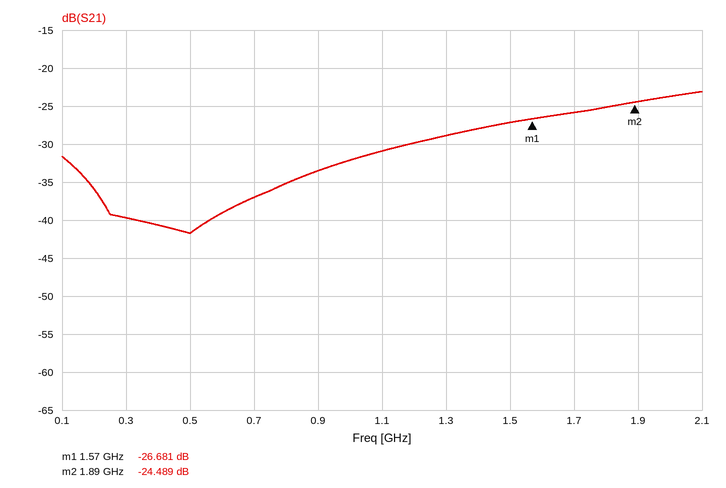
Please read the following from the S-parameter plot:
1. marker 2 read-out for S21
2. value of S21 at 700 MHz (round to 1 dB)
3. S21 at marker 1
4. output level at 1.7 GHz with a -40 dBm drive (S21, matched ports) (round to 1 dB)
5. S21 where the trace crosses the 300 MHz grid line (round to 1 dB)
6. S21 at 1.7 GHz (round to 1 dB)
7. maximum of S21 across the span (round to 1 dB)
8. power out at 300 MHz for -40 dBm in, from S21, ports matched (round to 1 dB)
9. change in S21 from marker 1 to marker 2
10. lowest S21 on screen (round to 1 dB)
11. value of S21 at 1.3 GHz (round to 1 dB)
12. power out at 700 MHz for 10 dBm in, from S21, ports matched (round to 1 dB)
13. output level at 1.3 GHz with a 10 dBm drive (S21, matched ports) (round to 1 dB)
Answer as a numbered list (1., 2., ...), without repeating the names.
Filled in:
1. -24.489 dB
2. -37 dB
3. -26.681 dB
4. -66 dBm
5. -40 dB
6. -26 dB
7. -23 dB
8. -80 dBm
9. 2.192 dB
10. -42 dB
11. -29 dB
12. -27 dBm
13. -19 dBm
